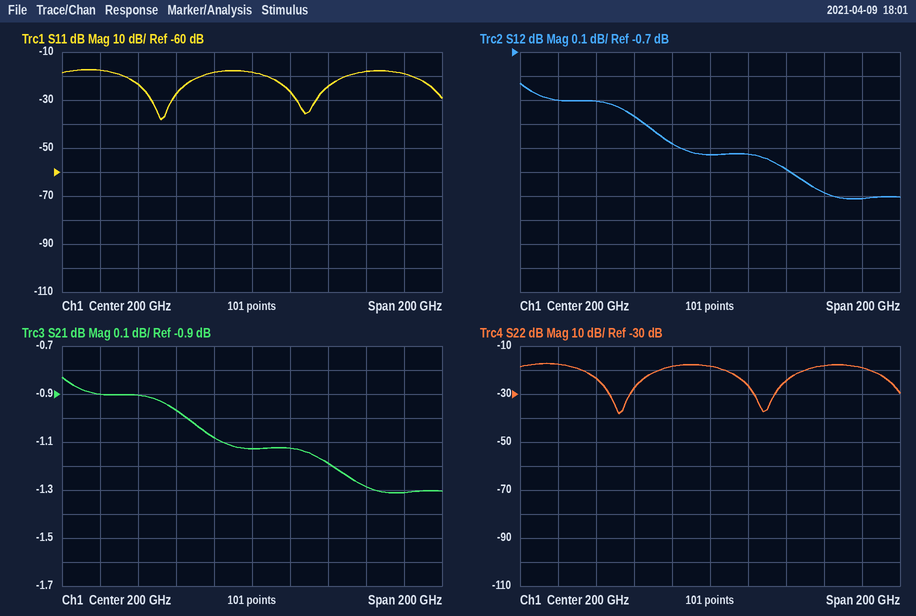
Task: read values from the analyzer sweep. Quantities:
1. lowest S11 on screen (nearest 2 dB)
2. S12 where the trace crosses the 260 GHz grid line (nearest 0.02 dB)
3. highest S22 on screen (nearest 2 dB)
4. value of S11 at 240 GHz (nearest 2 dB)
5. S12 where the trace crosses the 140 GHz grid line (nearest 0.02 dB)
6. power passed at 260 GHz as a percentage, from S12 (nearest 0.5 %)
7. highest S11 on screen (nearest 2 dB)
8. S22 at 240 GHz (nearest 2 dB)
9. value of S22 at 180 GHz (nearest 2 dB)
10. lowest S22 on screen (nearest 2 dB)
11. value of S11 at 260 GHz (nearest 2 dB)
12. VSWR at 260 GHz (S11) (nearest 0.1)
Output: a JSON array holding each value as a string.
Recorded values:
["-38 dB", "-1.28 dB", "-18 dB", "-24 dB", "-0.90 dB", "74.5 %", "-18 dB", "-24 dB", "-18 dB", "-38 dB", "-18 dB", "1.3"]
